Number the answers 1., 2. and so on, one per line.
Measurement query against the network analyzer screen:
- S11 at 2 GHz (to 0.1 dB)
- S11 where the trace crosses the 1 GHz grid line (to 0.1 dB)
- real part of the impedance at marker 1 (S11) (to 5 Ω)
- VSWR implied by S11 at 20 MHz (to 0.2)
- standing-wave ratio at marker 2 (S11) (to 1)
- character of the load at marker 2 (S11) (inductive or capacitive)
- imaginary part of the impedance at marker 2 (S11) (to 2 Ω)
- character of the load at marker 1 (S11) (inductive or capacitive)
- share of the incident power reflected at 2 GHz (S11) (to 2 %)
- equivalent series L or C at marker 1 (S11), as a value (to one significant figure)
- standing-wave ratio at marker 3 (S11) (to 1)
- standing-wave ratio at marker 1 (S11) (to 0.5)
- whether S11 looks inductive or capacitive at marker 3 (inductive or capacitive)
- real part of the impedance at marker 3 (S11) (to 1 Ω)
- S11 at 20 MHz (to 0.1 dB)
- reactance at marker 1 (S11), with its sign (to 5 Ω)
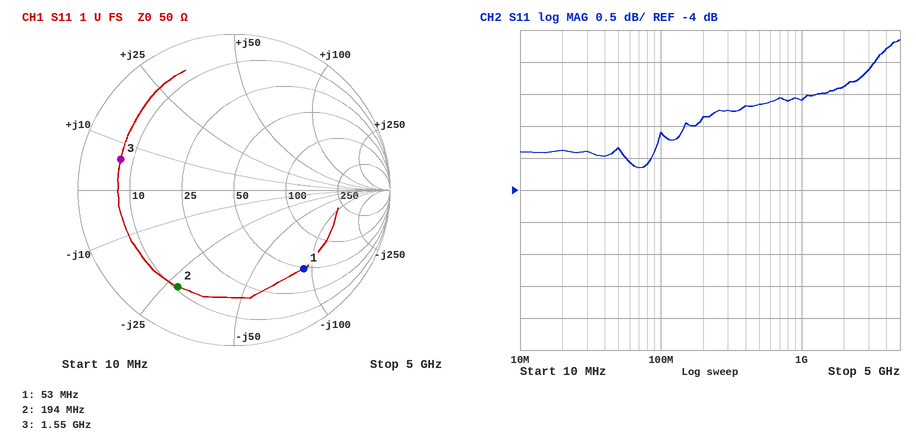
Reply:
1. -2.4 dB
2. -2.6 dB
3. 50 Ω
4. 5.2
5. 6
6. capacitive
7. -28 Ω
8. capacitive
9. 58 %
10. 30 pF
11. 7
12. 5.0
13. inductive
14. 7 Ω
15. -3.4 dB
16. -90 Ω
